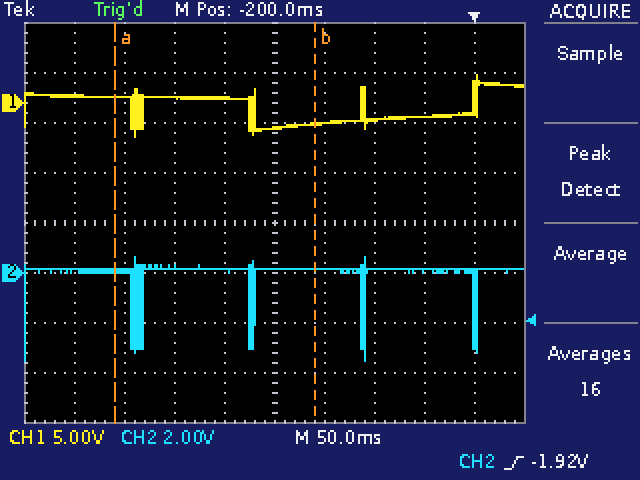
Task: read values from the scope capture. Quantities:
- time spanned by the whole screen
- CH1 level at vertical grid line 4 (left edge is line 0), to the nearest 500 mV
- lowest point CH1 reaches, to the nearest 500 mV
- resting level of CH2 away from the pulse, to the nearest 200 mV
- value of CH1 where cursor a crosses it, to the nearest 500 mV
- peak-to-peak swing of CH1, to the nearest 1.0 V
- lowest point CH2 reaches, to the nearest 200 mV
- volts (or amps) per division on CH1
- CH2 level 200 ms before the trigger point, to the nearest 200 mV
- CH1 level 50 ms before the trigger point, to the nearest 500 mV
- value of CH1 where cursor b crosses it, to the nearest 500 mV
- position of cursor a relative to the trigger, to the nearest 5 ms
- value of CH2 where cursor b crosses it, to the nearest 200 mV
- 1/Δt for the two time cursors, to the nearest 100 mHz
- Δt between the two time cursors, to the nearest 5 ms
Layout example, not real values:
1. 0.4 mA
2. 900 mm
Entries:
1. 500 ms
2. 500 mV
3. -3.5 V
4. 200 mV
5. 500 mV
6. 6.0 V
7. -3.6 V
8. 5 V
9. 200 mV
10. -1.5 V
11. -2.0 V
12. -360 ms
13. 200 mV
14. 5.0 Hz
15. 200 ms
